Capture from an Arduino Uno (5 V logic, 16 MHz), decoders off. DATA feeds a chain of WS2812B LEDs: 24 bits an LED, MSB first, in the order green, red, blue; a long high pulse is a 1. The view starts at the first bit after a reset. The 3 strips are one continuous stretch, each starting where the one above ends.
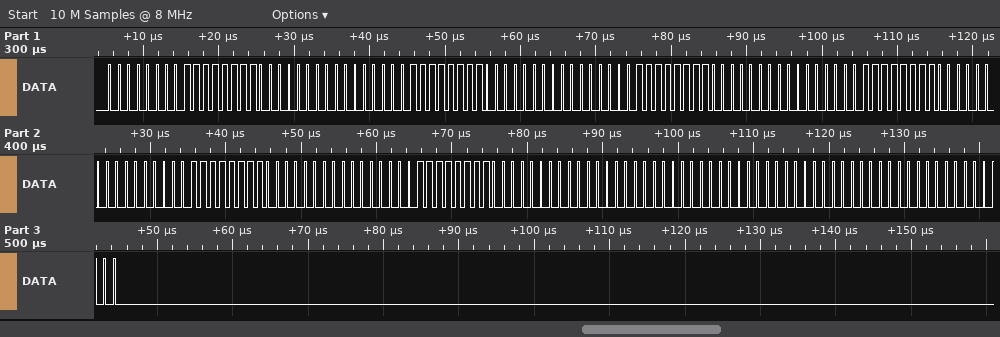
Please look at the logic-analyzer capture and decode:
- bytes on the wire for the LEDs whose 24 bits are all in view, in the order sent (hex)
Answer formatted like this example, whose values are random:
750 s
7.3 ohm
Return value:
00 FF 00 00 FF 00 00 FF 00 00 FF 00 00 FF 00 00 FF 00 00 00 00 00 00 00
